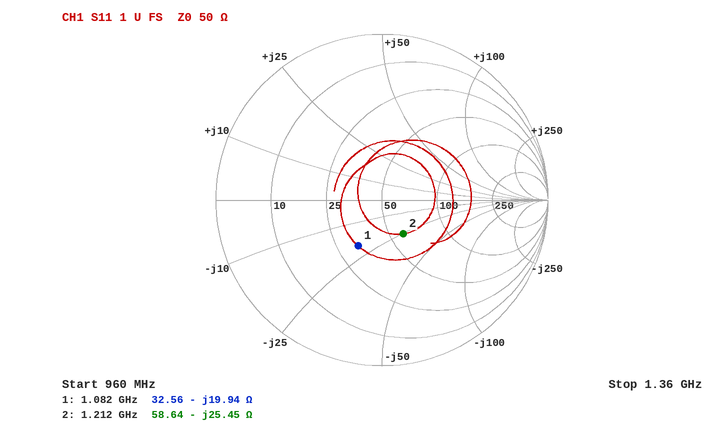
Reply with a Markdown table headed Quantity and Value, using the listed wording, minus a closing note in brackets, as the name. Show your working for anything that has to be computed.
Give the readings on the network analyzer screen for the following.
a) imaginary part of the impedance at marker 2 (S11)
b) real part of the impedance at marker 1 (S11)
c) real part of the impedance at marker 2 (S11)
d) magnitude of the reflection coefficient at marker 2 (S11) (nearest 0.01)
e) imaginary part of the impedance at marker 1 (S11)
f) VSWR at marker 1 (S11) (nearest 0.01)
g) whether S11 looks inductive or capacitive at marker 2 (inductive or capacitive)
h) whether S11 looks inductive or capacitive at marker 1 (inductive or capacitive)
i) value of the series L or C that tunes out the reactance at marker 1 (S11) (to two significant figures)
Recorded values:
| Quantity | Value |
|---|---|
| imaginary part of the impedance at marker 2 | -25.45 Ω |
| real part of the impedance at marker 1 | 32.56 Ω |
| real part of the impedance at marker 2 | 58.64 Ω |
| magnitude of the reflection coefficient at marker 2 (S11) | 0.24 |
| imaginary part of the impedance at marker 1 | -19.94 Ω |
| VSWR at marker 1 (S11) | 1.91 |
| whether S11 looks inductive or capacitive at marker 2 | capacitive |
| whether S11 looks inductive or capacitive at marker 1 | capacitive |
| value of the series L or C that tunes out the reactance at marker 1 (S11) | L = 19.94 Ω/(2π × 1.082 GHz) ≈ 2.9 nH |
